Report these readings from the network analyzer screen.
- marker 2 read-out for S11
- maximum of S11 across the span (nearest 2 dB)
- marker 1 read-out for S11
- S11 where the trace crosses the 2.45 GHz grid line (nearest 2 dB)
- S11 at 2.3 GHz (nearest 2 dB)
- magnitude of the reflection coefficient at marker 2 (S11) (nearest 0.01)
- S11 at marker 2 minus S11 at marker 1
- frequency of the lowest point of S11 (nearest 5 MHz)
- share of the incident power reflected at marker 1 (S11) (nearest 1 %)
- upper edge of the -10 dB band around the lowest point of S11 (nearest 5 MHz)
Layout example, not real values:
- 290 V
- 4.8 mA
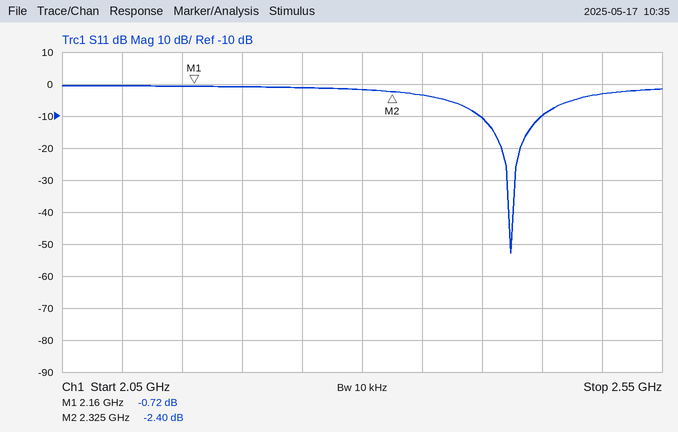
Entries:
- -2.40 dB
- 0 dB
- -0.72 dB
- -10 dB
- -2 dB
- 0.76
- -1.68 dB
- 2.425 GHz
- 85 %
- 2.450 GHz
